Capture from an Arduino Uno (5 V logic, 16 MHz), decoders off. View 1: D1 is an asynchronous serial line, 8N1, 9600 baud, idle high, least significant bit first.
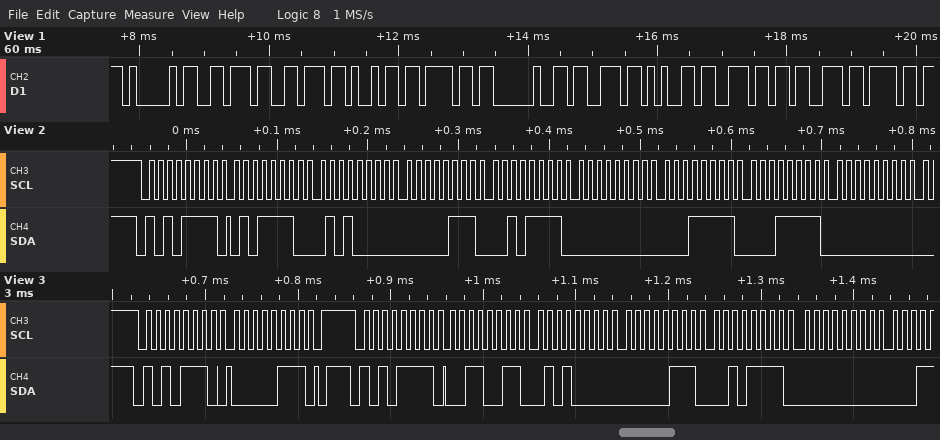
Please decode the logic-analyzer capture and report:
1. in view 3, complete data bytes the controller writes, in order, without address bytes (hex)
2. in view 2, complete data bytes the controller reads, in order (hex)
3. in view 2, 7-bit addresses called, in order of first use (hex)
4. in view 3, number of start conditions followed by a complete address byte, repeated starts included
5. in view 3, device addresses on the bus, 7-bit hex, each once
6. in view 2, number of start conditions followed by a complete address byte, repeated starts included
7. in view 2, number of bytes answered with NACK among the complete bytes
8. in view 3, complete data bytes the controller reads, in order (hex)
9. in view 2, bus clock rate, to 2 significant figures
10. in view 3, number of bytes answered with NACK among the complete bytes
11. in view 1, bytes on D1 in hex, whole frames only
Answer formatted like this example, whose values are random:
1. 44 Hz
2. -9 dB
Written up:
1. 07
2. 5E 50 07 2F 00 1F 1F 00
3. 0x57
4. 2
5. 0x57
6. 1
7. 0
8. 33 50 07 2F 00
9. 100 kHz
10. 0
11. 41 76 76 69 6F 20 73 65 6E 73 6F
